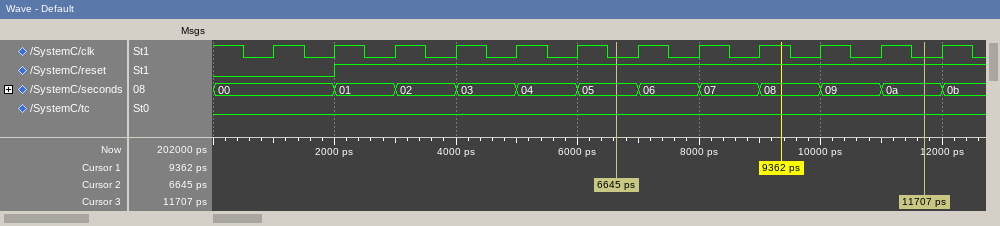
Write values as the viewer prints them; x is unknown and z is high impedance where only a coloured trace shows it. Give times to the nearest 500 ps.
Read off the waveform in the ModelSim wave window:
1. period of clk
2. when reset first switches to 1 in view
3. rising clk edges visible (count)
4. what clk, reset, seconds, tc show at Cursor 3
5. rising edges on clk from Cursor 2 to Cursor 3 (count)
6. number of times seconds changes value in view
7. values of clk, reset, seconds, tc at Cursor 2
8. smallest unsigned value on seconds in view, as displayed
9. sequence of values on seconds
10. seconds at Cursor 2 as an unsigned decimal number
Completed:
1000 ps
2000 ps
12
clk=0, reset=1, seconds=0a, tc=0
5
11
clk=0, reset=1, seconds=05, tc=0
00
00, 01, 02, 03, 04, 05, 06, 07, 08, 09, 0a, 0b
5
